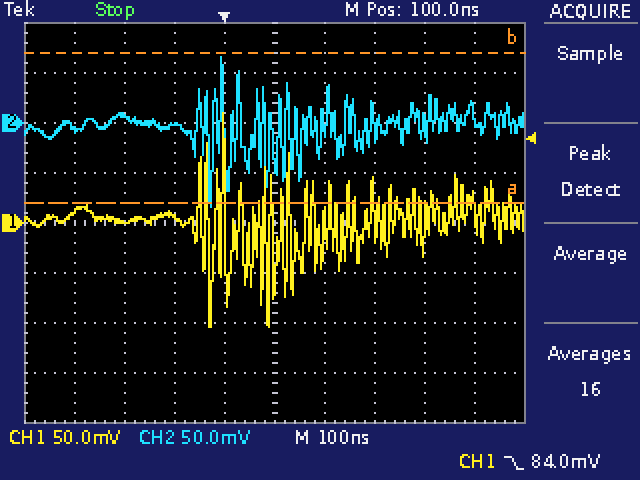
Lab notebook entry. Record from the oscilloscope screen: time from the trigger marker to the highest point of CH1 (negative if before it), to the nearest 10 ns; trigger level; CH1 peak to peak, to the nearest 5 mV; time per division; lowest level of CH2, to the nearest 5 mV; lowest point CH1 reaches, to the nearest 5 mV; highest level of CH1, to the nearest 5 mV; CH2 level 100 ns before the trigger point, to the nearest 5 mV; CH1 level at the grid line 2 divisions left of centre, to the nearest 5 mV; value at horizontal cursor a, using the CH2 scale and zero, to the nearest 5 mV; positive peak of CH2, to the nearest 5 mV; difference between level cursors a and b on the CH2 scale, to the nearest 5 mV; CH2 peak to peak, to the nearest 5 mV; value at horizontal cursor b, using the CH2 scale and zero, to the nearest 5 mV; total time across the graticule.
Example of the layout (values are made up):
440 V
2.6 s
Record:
0 ns
84.0 mV
215 mV
100 ns
-85 mV
-105 mV
110 mV
0 mV
5 mV
-80 mV
65 mV
150 mV
150 mV
70 mV
1 µs
